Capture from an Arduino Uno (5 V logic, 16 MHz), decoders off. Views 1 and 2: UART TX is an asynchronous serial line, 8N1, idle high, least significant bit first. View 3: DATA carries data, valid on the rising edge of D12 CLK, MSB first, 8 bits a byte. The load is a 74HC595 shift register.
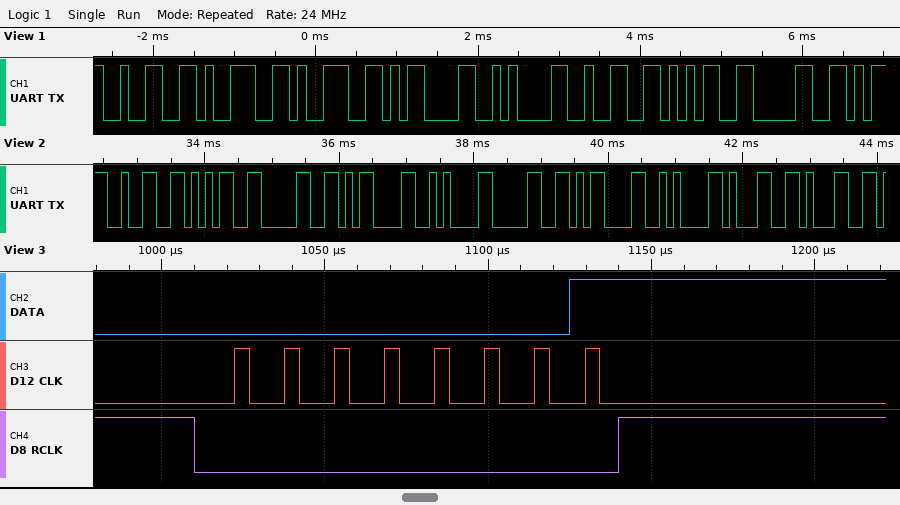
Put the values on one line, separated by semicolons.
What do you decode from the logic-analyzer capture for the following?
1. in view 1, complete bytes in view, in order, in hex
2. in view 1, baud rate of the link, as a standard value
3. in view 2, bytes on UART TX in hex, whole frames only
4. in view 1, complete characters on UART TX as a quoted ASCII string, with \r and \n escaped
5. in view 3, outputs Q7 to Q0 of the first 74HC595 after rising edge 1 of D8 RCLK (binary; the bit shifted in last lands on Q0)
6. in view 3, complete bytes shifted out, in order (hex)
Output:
32 39 39 0D 0A 32 35 30; 9600 baud; 32 35 30 0D 0A 30 0D 0A 31 31; "299\r\n250"; 00000001; 01
